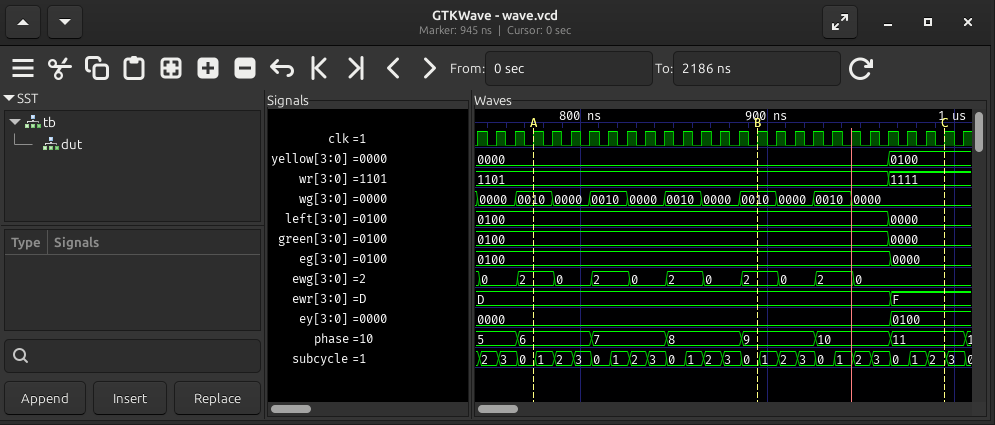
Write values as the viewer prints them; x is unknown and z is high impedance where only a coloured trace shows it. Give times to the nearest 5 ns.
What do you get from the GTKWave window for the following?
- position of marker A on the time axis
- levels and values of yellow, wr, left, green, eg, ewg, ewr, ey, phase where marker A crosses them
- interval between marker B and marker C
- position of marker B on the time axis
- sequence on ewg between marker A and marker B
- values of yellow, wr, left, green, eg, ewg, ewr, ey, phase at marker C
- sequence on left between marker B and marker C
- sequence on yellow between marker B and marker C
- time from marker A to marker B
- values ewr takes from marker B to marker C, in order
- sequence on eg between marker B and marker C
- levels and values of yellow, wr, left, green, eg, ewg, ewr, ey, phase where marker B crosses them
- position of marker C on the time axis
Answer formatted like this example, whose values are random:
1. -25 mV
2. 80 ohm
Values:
1. 775 ns
2. yellow=0000, wr=1101, left=0100, green=0100, eg=0100, ewg=2, ewr=D, ey=0000, phase=6
3. 100 ns
4. 895 ns
5. 2, 0, 2, 0, 2, 0, 2
6. yellow=0100, wr=1111, left=0000, green=0000, eg=0000, ewg=0, ewr=F, ey=0100, phase=11
7. 0100, 0000
8. 0000, 0100
9. 120 ns
10. D, F
11. 0100, 0000
12. yellow=0000, wr=1101, left=0100, green=0100, eg=0100, ewg=2, ewr=D, ey=0000, phase=9
13. 995 ns
